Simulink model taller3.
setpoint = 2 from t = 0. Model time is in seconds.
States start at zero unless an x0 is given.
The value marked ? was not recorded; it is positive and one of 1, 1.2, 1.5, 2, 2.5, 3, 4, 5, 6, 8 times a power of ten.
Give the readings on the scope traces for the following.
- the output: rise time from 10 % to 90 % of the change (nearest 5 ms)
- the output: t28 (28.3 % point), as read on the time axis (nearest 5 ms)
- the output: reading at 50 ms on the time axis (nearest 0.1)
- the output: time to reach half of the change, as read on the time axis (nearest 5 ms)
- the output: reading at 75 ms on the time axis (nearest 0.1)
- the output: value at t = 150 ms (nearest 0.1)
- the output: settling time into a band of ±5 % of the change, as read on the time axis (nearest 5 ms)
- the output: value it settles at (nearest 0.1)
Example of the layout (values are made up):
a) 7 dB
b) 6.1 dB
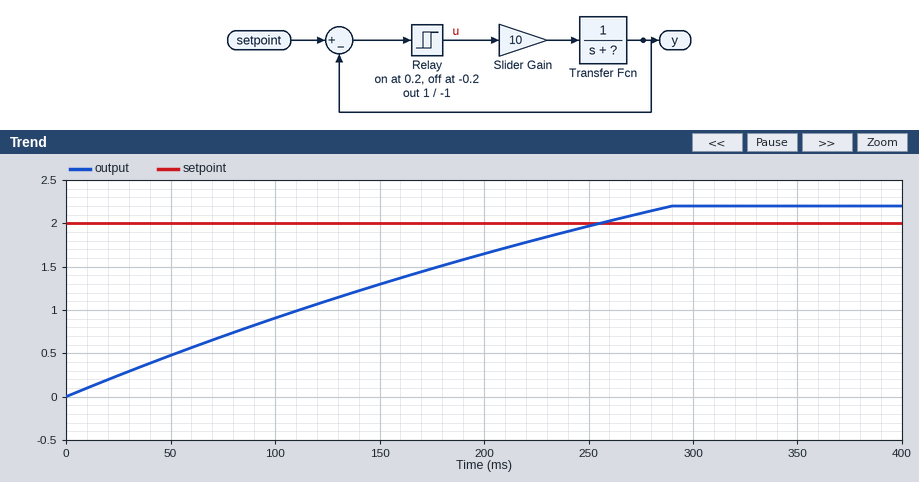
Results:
a) 230 ms
b) 65 ms
c) 0.5
d) 125 ms
e) 0.7
f) 1.3
g) 270 ms
h) 2.2
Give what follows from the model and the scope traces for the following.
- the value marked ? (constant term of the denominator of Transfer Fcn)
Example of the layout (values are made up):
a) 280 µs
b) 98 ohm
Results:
a) 2
